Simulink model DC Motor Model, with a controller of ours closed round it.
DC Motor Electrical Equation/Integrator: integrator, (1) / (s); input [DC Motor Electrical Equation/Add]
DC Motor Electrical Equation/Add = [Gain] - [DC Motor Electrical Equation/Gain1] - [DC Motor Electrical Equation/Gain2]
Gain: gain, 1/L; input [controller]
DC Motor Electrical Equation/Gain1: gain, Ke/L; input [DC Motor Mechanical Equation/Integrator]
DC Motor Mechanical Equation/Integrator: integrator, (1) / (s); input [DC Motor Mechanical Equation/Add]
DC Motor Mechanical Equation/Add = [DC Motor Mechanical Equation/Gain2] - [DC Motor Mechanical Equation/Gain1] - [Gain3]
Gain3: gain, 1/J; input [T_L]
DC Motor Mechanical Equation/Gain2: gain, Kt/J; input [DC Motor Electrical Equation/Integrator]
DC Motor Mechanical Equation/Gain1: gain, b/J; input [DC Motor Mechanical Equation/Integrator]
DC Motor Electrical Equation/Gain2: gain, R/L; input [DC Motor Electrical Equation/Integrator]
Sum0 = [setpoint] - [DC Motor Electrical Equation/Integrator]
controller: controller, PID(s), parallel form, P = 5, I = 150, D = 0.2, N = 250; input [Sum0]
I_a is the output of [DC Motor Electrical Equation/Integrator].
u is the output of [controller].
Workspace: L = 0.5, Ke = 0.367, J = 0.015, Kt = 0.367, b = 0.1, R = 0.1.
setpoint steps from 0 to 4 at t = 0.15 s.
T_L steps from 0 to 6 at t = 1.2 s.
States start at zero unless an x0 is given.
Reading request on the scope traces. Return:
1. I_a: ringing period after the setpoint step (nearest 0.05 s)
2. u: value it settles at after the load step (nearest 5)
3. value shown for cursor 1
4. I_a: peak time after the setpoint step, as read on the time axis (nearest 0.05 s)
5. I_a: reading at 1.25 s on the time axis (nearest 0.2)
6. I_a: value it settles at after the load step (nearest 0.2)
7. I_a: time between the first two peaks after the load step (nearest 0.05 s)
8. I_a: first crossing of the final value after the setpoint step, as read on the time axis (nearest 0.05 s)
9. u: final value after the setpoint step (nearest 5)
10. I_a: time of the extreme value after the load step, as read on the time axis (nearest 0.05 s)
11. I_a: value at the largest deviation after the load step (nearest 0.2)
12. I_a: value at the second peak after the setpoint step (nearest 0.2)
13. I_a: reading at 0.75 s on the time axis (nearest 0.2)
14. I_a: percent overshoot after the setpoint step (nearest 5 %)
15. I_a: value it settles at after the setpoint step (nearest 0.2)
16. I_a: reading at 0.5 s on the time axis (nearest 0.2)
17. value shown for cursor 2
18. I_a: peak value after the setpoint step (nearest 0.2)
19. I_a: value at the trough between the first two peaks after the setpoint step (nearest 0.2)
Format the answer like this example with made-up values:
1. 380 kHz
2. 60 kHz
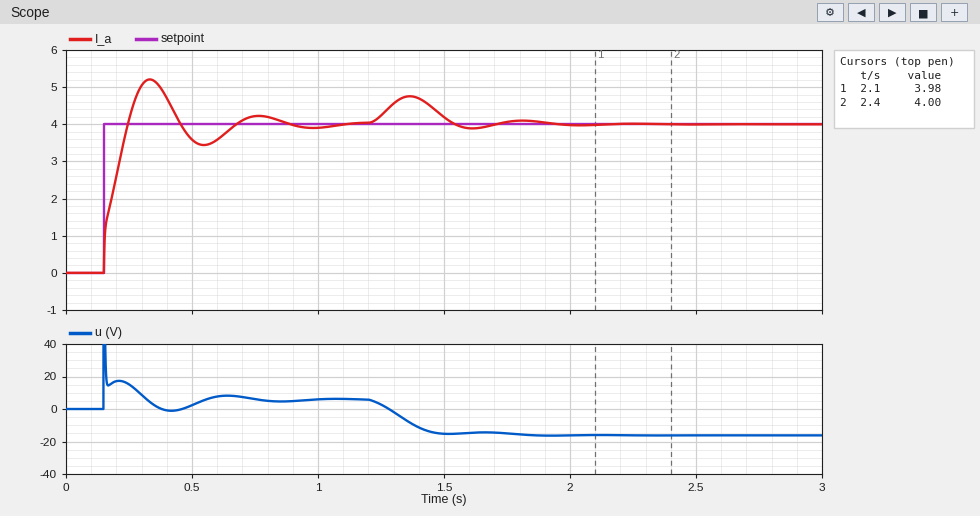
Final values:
1. 0.45 s
2. -15
3. 3.98
4. 0.35 s
5. 4.2
6. 4.0
7. 0.45 s
8. 0.25 s
9. 5
10. 1.35 s
11. 4.8
12. 4.2
13. 4.2
14. 30 %
15. 4.0
16. 3.6
17. 4.00
18. 5.2
19. 3.4
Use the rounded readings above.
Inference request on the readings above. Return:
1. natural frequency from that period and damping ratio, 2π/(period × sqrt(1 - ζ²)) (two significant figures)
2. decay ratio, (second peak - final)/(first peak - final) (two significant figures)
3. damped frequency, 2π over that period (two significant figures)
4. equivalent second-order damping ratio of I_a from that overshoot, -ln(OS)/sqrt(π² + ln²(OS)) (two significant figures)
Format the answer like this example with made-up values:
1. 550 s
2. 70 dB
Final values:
1. 15 rad/s
2. 0.17
3. 14 rad/s
4. 0.36
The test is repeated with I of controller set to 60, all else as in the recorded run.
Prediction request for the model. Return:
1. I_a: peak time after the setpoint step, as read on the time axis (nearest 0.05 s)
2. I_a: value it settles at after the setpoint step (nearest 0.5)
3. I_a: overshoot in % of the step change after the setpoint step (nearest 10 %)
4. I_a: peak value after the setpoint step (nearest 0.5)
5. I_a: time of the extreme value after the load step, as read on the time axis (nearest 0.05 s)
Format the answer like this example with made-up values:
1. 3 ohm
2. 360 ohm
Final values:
1. 0.40 s
2. 4.0
3. 20 %
4. 4.5
5. 1.45 s
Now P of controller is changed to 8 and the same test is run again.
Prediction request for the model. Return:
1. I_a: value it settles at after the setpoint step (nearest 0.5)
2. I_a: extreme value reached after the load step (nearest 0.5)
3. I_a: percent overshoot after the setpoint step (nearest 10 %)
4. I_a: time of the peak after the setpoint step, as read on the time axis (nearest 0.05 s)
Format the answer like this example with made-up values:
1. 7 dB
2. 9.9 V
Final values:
1. 4.0
2. 4.5
3. 20 %
4. 0.30 s
